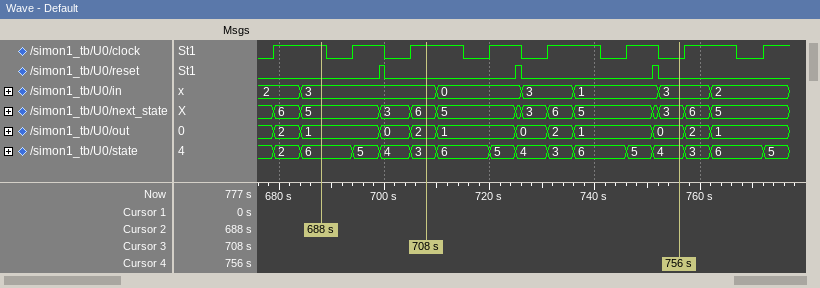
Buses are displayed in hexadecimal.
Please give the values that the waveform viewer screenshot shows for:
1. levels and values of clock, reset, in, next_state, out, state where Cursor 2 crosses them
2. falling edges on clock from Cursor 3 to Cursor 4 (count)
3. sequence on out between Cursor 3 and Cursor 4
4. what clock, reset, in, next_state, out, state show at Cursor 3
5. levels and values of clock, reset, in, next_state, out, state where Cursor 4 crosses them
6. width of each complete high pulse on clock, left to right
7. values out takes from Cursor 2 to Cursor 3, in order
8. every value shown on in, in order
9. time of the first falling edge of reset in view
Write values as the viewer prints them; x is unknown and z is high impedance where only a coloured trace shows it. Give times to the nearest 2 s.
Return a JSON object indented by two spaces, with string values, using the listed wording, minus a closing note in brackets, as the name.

{
  "levels and values of clock, reset, in, next_state, out, state where Cursor 2 crosses them": "clock=1, reset=0, in=3, next_state=5, out=1, state=6",
  "falling edges on clock from Cursor 3 to Cursor 4": "4",
  "sequence on out between Cursor 3 and Cursor 4": "2, 1, 0, 2, 1, 0",
  "what clock, reset, in, next_state, out, state show at Cursor 3": "clock=1, reset=0, in=3, next_state=6, out=2, state=3",
  "levels and values of clock, reset, in, next_state, out, state where Cursor 4 crosses them": "clock=0, reset=0, in=3, next_state=3, out=0, state=4",
  "width of each complete high pulse on clock, left to right": "10 s, 6 s, 10 s, 6 s, 10 s, 6 s, 10 s",
  "values out takes from Cursor 2 to Cursor 3, in order": "1, 0, 2",
  "every value shown on in, in order": "2, 3, 0, 3, 1, 3, 2",
  "time of the first falling edge of reset in view": "700 s"
}
